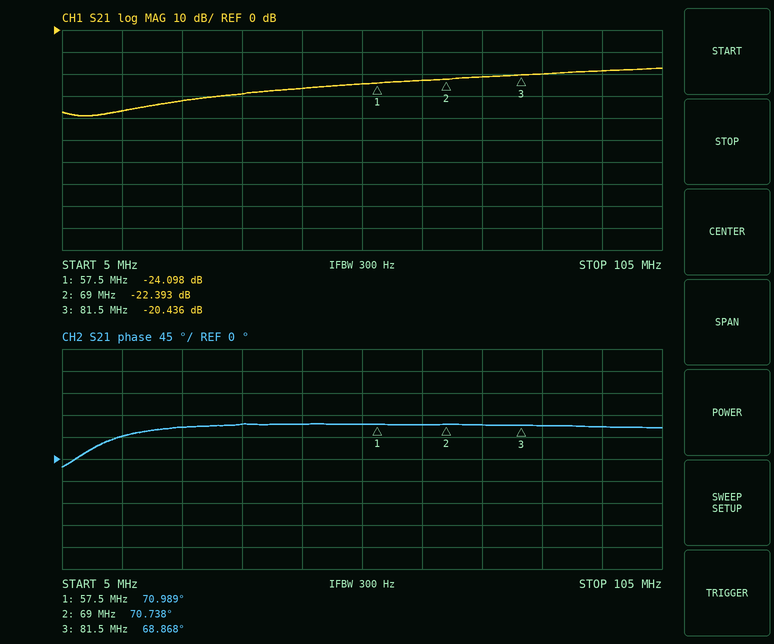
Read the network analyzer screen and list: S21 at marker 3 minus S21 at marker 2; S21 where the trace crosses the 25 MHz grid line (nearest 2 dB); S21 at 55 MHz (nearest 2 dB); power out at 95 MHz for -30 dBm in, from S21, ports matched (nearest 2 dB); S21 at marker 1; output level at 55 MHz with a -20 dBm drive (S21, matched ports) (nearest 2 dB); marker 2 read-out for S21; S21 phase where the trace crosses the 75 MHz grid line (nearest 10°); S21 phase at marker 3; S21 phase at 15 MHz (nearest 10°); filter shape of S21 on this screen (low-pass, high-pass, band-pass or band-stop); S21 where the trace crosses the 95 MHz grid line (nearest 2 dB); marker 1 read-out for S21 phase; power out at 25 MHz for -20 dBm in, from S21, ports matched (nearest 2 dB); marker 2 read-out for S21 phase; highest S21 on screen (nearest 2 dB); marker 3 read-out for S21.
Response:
1.957 dB
-32 dB
-24 dB
-48 dBm
-24.098 dB
-44 dBm
-22.393 dB
70°
68.868°
50°
high-pass
-18 dB
70.989°
-52 dBm
70.738°
-18 dB
-20.436 dB
